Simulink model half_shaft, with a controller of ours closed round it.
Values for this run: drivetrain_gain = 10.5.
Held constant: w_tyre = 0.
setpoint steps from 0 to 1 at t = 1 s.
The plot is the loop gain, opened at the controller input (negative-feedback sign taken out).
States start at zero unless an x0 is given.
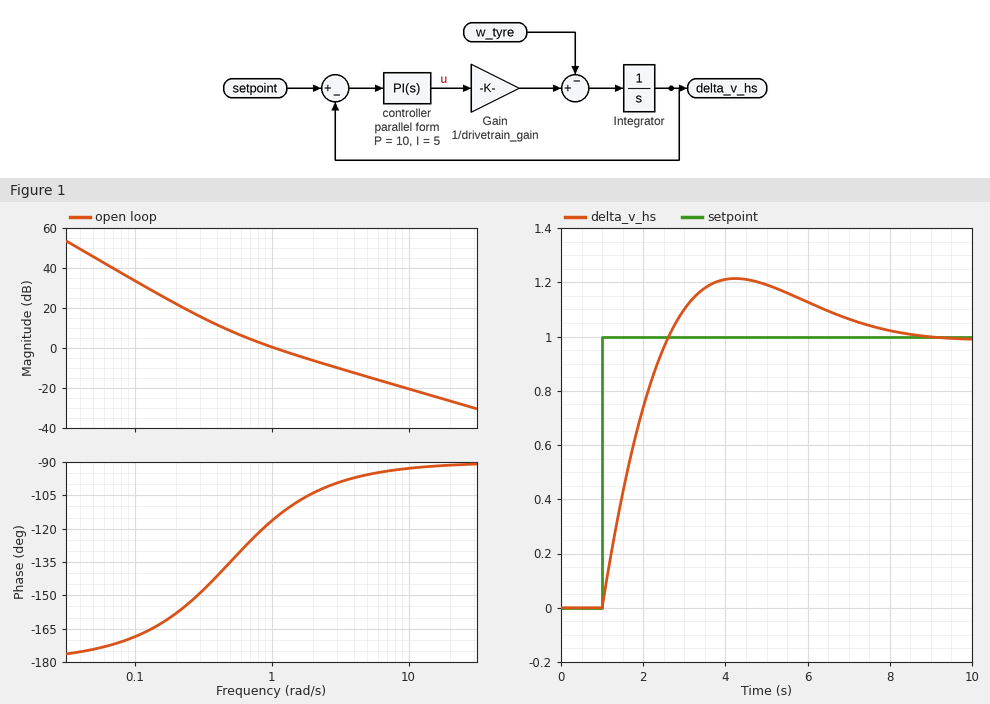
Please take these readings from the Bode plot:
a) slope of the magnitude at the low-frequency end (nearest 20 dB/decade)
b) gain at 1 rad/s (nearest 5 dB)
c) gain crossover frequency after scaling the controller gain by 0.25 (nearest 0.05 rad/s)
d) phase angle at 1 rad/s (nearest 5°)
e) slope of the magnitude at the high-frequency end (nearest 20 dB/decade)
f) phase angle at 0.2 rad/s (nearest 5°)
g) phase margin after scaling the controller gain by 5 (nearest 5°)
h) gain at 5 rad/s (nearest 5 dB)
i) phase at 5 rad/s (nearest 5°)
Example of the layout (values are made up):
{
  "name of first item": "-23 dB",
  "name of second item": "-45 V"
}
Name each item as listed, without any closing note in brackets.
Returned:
{
  "slope of the magnitude at the low-frequency end": "-40 dB/decade",
  "gain at 1 rad/s": "0 dB",
  "gain crossover frequency after scaling the controller gain by 0.25": "0.40 rad/s",
  "phase angle at 1 rad/s": "-115°",
  "slope of the magnitude at the high-frequency end": "-20 dB/decade",
  "phase angle at 0.2 rad/s": "-160°",
  "phase margin after scaling the controller gain by 5": "85°",
  "gain at 5 rad/s": "-15 dB",
  "phase at 5 rad/s": "-95°"
}
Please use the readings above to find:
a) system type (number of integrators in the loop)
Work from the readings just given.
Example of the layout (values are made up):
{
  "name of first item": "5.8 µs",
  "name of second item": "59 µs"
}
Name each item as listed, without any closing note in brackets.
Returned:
{
  "system type": "2"
}
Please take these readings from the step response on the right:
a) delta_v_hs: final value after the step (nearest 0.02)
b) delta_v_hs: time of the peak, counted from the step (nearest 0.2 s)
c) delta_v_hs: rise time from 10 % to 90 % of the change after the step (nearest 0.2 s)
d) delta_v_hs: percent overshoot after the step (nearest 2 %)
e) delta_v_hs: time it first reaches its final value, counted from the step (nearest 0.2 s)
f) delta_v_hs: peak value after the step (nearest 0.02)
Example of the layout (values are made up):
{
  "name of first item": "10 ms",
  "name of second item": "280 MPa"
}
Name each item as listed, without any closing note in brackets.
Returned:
{
  "delta_v_hs: final value after the step": "1.00",
  "delta_v_hs: time of the peak, counted from the step": "3.2 s",
  "delta_v_hs: rise time from 10 % to 90 % of the change after the step": "1.2 s",
  "delta_v_hs: percent overshoot after the step": "22 %",
  "delta_v_hs: time it first reaches its final value, counted from the step": "1.6 s",
  "delta_v_hs: peak value after the step": "1.22"
}
